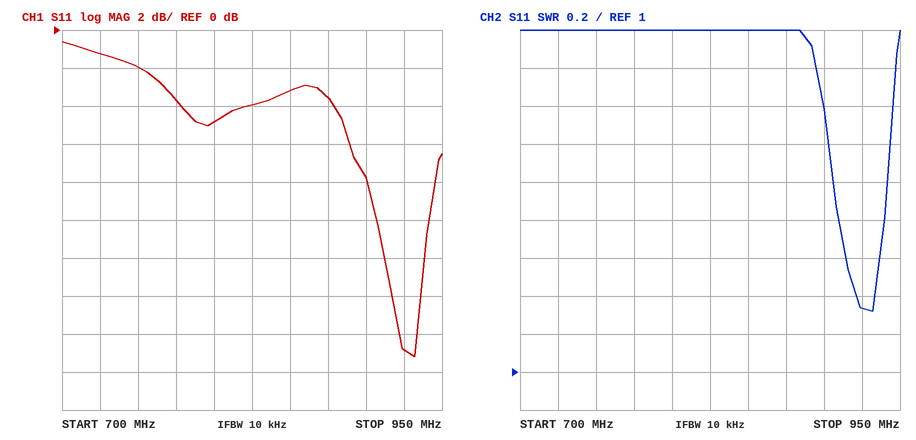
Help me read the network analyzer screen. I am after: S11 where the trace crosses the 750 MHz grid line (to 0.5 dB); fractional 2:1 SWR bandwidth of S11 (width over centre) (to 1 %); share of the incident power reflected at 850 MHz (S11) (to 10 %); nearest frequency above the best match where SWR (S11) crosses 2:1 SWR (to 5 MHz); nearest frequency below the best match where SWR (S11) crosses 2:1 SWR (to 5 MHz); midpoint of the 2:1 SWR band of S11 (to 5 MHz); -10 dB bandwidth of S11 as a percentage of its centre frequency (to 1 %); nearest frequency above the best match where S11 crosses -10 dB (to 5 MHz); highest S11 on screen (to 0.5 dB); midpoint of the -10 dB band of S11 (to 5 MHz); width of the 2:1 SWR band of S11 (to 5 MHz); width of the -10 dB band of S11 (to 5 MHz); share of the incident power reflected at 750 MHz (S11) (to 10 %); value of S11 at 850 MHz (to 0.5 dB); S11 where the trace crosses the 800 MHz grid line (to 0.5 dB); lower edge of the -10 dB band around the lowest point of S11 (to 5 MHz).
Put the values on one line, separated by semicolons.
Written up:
-2.0 dB; 4 %; 50 %; 940 MHz; 905 MHz; 925 MHz; 4 %; 940 MHz; -0.5 dB; 925 MHz; 35 MHz; 35 MHz; 60 %; -3.0 dB; -5.0 dB; 905 MHz
